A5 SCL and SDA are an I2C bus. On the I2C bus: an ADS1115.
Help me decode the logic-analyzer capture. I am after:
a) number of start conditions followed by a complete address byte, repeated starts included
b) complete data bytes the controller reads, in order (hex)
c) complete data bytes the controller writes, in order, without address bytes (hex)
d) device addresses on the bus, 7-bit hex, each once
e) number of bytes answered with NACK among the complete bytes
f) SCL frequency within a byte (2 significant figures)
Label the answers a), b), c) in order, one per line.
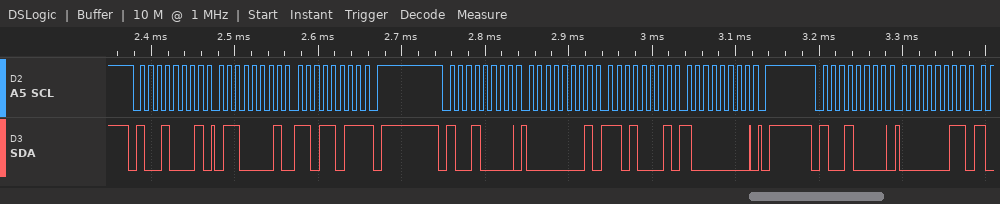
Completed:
a) 3
b) 61 DB
c) 01 D1 80 03
d) 0x48
e) 1
f) 100 kHz
